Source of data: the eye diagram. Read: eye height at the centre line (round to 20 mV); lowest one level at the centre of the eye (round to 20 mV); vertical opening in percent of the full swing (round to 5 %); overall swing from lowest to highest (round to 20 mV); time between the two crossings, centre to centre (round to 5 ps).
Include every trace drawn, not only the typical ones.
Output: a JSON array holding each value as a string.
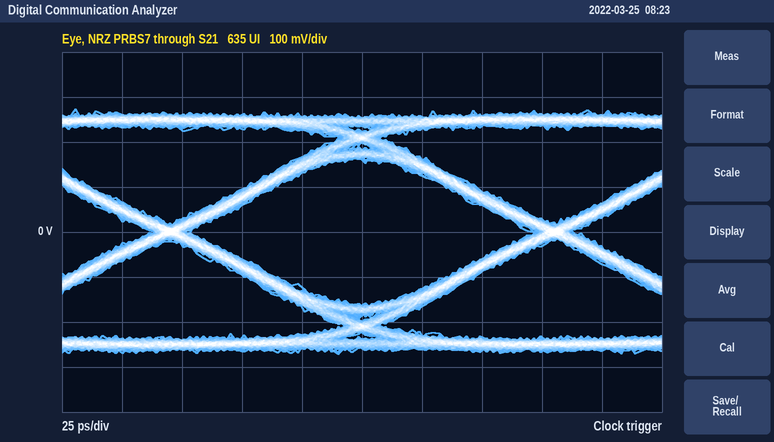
["320 mV", "160 mV", "60 %", "540 mV", "160 ps"]
